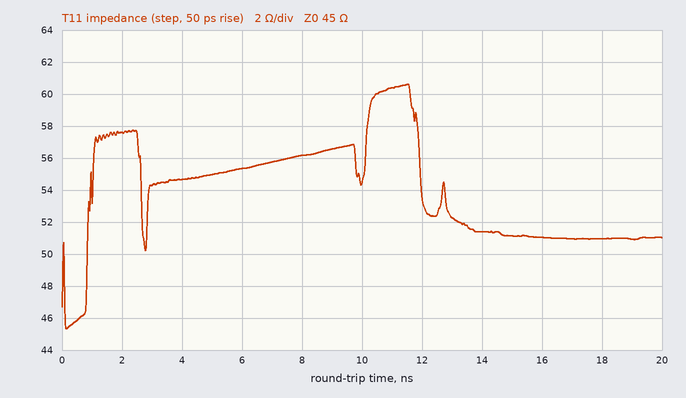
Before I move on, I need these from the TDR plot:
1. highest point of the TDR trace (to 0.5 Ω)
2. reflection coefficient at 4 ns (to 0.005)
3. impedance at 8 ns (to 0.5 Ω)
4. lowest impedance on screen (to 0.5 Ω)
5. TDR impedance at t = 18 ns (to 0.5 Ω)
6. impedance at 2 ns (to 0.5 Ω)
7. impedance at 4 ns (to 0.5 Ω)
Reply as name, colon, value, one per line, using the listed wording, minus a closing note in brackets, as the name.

highest point of the TDR trace: 60.5 Ω
reflection coefficient at 4 ns: +0.095
impedance at 8 ns: 56.0 Ω
lowest impedance on screen: 45.5 Ω
TDR impedance at t = 18 ns: 51.0 Ω
impedance at 2 ns: 57.5 Ω
impedance at 4 ns: 54.5 Ω
